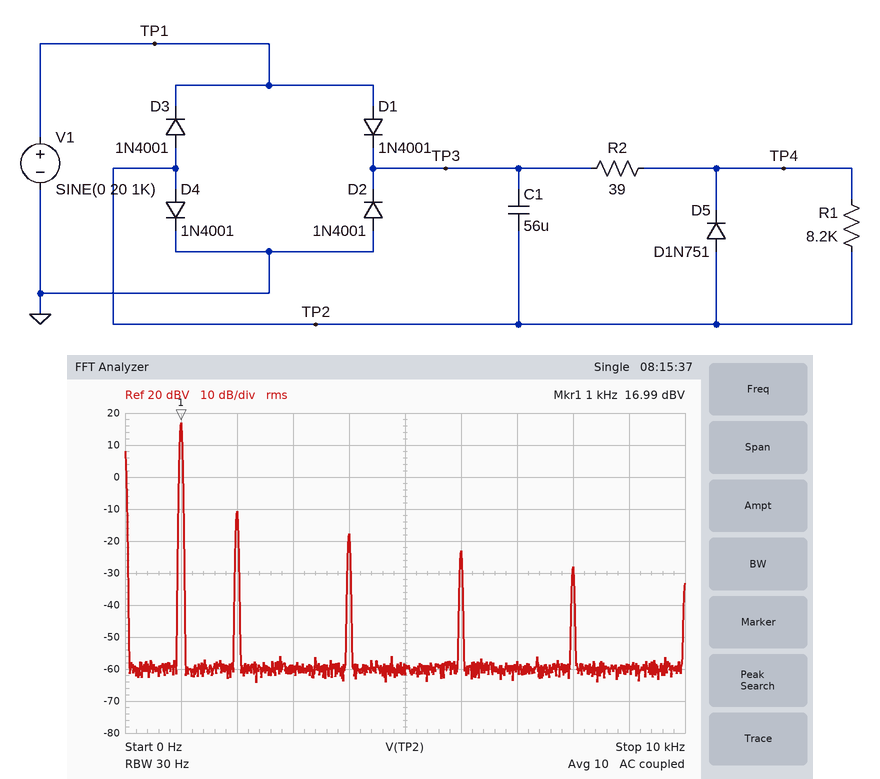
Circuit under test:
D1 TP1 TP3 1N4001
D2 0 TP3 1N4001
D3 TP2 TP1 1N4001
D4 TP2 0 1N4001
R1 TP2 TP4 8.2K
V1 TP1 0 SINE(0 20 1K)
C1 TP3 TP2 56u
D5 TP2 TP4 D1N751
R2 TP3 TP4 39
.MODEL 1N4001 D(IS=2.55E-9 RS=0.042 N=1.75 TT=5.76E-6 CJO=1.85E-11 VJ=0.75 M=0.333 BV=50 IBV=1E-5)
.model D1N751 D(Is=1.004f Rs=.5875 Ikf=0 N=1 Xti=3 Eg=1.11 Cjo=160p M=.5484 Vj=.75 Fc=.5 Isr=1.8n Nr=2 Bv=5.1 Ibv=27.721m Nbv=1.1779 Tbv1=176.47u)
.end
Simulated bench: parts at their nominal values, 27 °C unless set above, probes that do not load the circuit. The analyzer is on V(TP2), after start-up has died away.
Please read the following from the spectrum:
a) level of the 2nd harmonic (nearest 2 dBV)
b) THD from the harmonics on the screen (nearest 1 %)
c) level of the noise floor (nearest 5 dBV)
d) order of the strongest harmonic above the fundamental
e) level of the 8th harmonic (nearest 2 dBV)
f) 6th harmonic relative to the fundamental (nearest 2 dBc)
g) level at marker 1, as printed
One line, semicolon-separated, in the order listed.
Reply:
-10 dBV; 5 %; -60 dBV; 2; -28 dBV; -40 dBc; 16.99 dBV
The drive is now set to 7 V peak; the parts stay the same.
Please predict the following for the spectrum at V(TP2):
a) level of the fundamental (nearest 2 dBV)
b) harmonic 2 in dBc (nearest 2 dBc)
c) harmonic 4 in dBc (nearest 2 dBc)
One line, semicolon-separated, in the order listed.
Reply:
8 dBV; -50 dBc; -56 dBc
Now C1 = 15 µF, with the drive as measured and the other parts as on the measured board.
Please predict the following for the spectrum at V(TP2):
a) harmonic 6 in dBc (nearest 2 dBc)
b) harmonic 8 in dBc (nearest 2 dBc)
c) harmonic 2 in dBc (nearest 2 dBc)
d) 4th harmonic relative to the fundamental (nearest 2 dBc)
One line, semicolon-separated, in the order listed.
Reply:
-36 dBc; -44 dBc; -18 dBc; -28 dBc
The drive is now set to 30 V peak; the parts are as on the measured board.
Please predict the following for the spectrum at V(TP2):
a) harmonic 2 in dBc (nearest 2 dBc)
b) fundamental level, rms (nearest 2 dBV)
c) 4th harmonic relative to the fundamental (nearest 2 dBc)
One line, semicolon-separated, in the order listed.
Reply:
-26 dBc; 20 dBV; -34 dBc
